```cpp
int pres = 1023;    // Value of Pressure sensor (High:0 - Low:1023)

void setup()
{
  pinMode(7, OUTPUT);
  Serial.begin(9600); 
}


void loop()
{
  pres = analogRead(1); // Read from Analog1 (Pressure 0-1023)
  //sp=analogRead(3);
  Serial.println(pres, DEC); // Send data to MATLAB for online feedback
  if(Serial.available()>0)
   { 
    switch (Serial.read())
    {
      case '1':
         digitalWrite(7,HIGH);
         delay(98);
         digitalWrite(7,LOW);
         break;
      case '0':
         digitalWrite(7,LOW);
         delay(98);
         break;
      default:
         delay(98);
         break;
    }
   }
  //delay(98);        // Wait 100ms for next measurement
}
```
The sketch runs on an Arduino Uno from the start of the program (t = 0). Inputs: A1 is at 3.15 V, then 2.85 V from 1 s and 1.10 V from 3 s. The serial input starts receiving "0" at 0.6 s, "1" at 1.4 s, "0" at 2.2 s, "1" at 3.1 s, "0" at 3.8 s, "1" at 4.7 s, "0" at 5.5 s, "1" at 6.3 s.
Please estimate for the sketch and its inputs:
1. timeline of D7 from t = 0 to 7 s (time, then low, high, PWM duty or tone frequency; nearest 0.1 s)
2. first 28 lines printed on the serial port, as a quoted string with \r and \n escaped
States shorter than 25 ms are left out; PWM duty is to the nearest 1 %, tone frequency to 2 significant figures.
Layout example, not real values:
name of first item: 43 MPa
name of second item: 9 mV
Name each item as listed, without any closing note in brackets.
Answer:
timeline of D7 from t = 0 to 7 s: 0 s low; 1.4 s high; 1.5 s low; 3.1 s high; 3.2 s low; 4.7 s high; 4.8 s low; 6.3 s high; 6.4 s low
first 28 lines printed on the serial port, as a quoted string with \r and \n escaped: "645\r\n645\r\n645\r\n645\r\n645\r\n645\r\n645\r\n645\r\n645\r\n645\r\n645\r\n645\r\n645\r\n645\r\n645\r\n645\r\n645\r\n645\r\n645\r\n645\r\n645\r\n645\r\n645\r\n645\r\n645\r\n645\r\n645\r\n645\r\n"
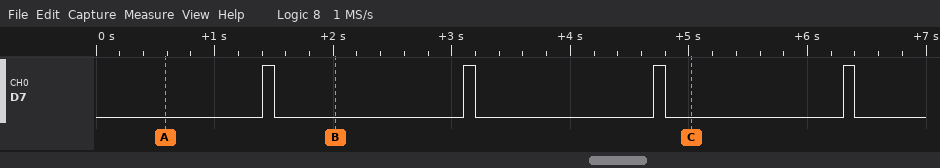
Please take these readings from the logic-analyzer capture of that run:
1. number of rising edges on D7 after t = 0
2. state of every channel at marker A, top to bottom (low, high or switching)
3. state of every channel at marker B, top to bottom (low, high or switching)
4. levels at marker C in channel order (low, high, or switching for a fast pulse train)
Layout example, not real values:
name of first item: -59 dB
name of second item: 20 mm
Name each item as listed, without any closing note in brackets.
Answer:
number of rising edges on D7 after t = 0: 4
state of every channel at marker A, top to bottom: D7 low
state of every channel at marker B, top to bottom: D7 low
levels at marker C in channel order: D7 low
